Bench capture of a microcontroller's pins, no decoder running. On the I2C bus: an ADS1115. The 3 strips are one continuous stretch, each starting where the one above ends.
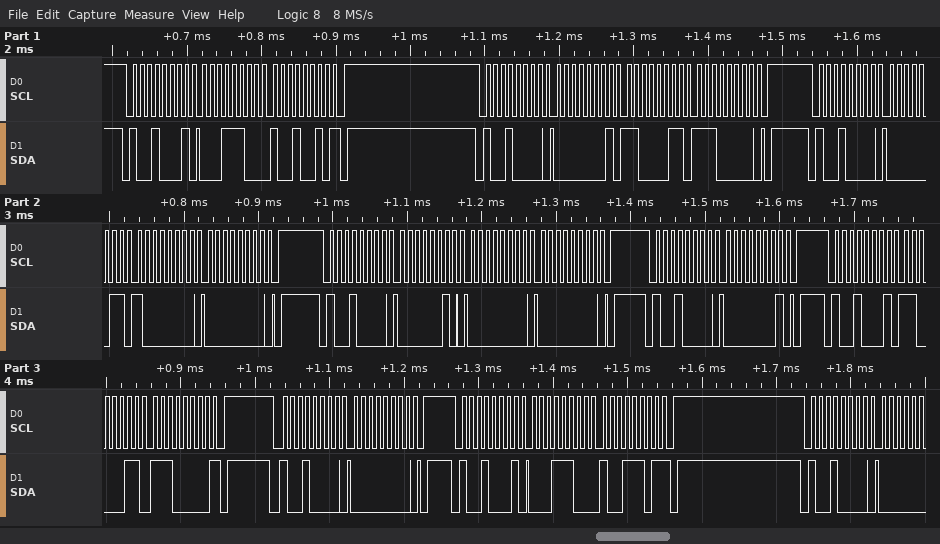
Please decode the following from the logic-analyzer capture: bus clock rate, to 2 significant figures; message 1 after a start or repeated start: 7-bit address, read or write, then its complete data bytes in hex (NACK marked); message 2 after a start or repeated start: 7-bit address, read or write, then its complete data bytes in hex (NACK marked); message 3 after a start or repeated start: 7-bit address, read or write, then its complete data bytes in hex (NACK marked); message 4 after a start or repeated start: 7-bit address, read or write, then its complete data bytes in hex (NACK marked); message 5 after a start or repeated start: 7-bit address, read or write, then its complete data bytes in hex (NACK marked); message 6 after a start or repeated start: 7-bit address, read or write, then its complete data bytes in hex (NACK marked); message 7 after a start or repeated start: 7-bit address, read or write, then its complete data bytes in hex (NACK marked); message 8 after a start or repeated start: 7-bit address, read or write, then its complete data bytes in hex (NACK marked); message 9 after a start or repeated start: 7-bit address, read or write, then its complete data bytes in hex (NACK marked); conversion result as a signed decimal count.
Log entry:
100 kHz
0x48 read: 1C 92 NACK
0x48 write: 01 C3 E0
0x48 write: 03 80 00
0x48 write: 02 00 00
0x48 write: 01
0x48 read: C3 E0 NACK
0x48 write: 00
0x48 read: 1C 9D NACK
0x48 write
7325
